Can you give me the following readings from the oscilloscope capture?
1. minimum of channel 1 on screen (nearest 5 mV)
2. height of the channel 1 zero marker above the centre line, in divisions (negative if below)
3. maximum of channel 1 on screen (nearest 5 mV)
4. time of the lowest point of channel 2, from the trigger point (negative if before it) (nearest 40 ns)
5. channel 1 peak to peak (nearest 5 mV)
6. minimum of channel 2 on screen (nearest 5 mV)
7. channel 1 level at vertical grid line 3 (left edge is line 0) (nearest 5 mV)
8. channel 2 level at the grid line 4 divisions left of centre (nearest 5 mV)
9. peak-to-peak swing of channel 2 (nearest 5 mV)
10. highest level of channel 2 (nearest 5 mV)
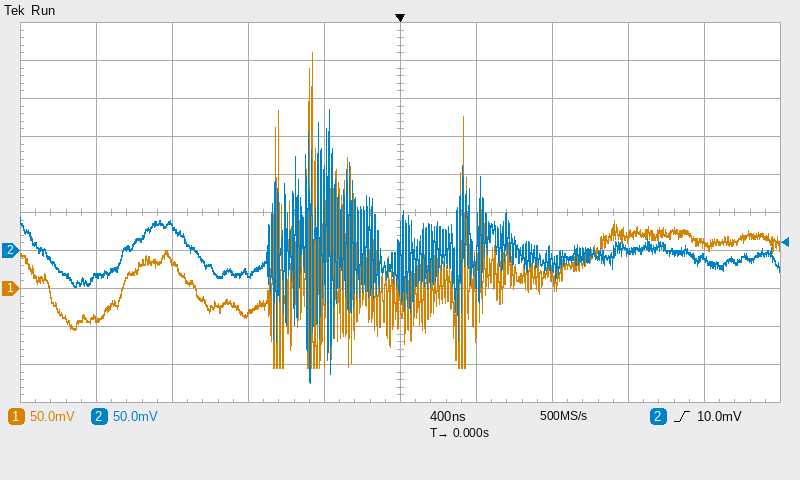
-105 mV
-2.0 div
310 mV
-480 ns
415 mV
-175 mV
-35 mV
-35 mV
360 mV
185 mV
